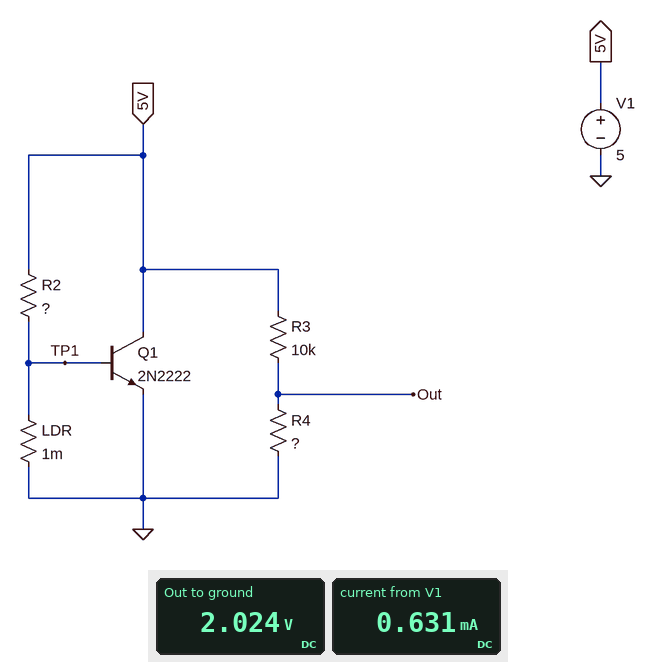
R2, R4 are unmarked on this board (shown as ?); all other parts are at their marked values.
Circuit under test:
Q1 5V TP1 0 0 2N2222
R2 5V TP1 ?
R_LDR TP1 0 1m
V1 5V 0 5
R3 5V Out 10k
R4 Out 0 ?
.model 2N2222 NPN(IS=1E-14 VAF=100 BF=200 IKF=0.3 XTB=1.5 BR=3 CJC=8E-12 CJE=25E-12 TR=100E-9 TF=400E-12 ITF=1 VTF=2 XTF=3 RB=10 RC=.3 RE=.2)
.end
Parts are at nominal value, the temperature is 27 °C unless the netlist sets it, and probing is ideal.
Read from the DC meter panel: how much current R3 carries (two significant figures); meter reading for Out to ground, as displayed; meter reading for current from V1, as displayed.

300 µA
2.024 V
0.631 mA
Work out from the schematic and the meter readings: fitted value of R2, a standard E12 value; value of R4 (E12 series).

15 kΩ
6.8 kΩ
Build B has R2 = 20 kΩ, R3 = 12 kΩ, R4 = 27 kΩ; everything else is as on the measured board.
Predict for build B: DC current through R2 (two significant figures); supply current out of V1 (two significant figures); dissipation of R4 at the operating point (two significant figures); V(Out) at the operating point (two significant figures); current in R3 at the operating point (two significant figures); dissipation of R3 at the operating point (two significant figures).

250 µA
380 µA
440 µW
3.5 V
130 µA
200 µW
